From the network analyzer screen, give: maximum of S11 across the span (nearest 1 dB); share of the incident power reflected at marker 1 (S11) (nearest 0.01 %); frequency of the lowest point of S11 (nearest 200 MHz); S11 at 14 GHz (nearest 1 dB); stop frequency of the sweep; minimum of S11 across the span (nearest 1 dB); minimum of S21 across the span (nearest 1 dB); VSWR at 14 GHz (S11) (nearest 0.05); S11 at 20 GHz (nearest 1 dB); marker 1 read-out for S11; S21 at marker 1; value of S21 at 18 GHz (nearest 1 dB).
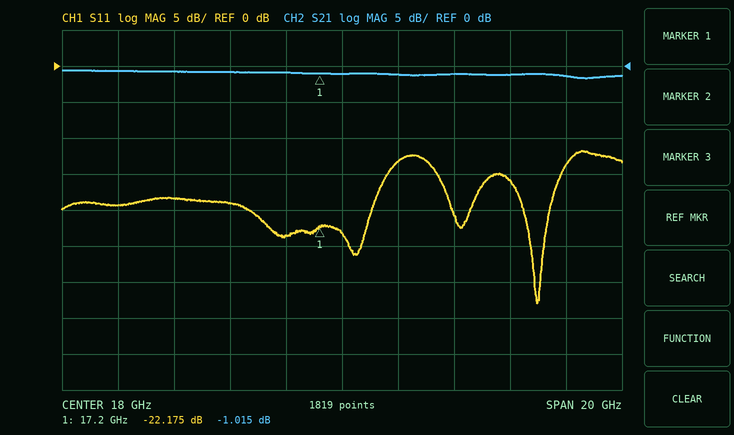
-12 dB
0.61 %
25.0 GHz
-19 dB
28 GHz
-33 dB
-2 dB
1.25
-13 dB
-22.175 dB
-1.015 dB
-1 dB
